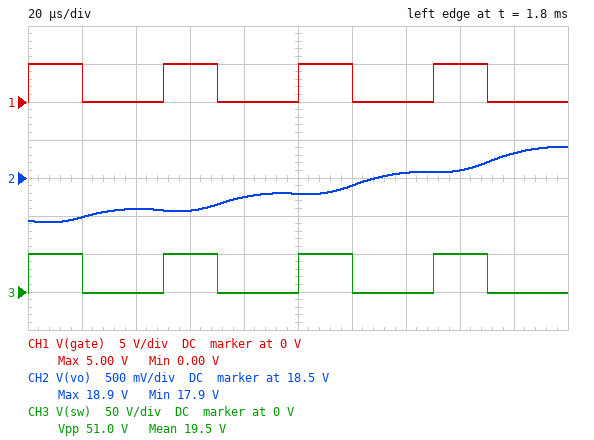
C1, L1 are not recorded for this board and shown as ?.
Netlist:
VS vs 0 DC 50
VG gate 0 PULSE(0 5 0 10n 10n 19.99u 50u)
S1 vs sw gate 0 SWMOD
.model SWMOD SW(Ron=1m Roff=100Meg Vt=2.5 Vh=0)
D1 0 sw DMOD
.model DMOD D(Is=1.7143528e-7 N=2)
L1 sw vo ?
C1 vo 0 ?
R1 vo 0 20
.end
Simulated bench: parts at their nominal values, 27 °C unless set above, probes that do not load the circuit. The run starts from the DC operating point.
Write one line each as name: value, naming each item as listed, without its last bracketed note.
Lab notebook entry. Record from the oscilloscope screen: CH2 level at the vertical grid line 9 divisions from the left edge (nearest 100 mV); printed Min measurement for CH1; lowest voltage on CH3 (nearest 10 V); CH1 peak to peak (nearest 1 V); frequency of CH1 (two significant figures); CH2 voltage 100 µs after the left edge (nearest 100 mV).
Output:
CH2 level at the vertical grid line 9 divisions from the left edge: 18.8 V
printed Min measurement for CH1: 0.00 V
lowest voltage on CH3: 0 V
CH1 peak to peak: 5 V
frequency of CH1: 20 kHz
CH2 voltage 100 µs after the left edge: 18.3 V
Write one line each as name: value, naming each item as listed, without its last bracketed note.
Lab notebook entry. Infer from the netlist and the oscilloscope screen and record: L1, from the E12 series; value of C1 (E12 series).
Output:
L1, from the E12 series: 680 µH
value of C1: 56 µF
